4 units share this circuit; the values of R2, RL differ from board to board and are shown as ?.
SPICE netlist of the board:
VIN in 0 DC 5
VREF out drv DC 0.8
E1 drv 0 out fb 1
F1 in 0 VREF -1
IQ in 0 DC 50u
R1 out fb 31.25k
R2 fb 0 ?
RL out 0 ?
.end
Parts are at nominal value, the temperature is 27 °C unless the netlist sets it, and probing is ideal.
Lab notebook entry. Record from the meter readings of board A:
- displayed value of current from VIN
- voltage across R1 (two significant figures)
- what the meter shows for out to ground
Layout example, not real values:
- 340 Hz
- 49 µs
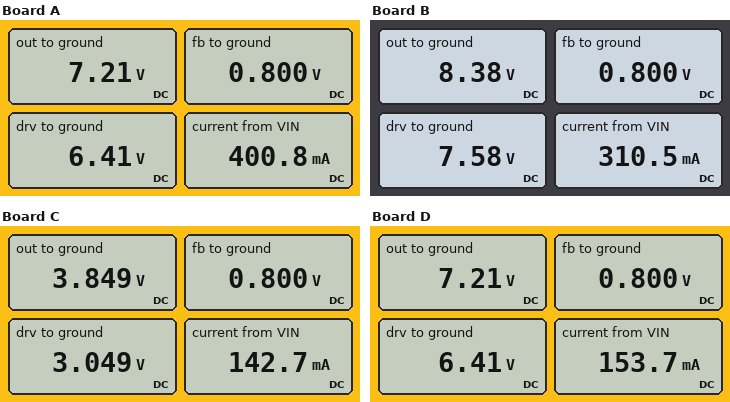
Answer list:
- 400.8 mA
- 6.4 V
- 7.21 V
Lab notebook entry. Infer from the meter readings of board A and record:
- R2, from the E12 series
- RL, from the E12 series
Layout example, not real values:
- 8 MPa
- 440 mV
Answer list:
- 3.9 kΩ
- 18 Ω
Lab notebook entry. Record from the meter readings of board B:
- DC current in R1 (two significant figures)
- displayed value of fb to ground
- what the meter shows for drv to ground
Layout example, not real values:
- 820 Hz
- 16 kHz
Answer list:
- 240 µA
- 0.800 V
- 7.58 V
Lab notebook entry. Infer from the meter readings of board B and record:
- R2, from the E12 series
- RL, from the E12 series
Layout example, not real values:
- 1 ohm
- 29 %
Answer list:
- 3.3 kΩ
- 27 Ω
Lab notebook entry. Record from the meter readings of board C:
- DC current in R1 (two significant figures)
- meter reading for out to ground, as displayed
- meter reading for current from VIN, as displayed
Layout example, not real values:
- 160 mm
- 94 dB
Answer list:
- 98 µA
- 3.849 V
- 142.7 mA
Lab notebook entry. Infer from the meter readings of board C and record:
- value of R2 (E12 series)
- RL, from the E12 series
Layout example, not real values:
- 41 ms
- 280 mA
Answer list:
- 8.2 kΩ
- 27 Ω
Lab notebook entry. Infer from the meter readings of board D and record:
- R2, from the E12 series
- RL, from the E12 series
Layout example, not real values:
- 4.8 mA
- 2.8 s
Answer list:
- 3.9 kΩ
- 47 Ω
